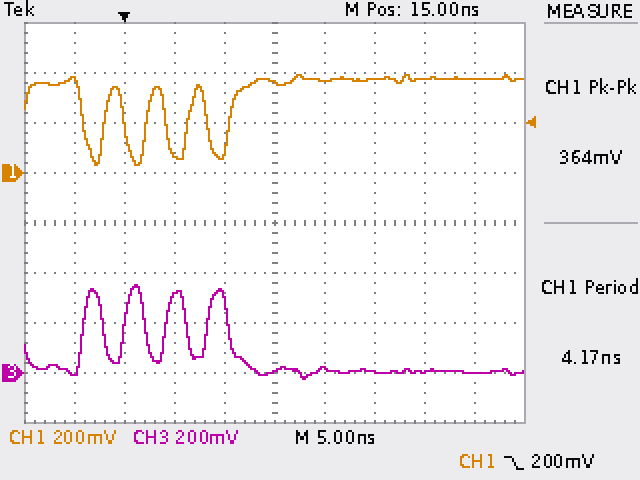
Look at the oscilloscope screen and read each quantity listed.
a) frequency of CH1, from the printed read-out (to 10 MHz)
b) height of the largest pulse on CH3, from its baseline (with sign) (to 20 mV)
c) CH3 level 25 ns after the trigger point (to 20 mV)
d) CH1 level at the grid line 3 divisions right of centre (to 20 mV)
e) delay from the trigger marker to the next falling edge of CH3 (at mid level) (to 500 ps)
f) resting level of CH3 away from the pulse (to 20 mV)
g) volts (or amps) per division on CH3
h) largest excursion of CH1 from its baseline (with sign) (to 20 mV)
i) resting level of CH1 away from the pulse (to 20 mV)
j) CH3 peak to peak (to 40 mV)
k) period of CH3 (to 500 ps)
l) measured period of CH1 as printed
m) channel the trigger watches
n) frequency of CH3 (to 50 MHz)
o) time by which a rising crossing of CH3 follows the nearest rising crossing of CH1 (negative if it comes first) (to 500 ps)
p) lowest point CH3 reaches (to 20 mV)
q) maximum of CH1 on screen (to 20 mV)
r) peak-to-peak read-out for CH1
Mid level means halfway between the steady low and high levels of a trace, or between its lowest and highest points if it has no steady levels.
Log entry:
240 MHz
+340 mV
0 mV
380 mV
2.0 ns
0 mV
200 mV
-340 mV
380 mV
360 mV
4.0 ns
4.17 ns
CH1
250 MHz
+2.0 ns
-20 mV
400 mV
364 mV
